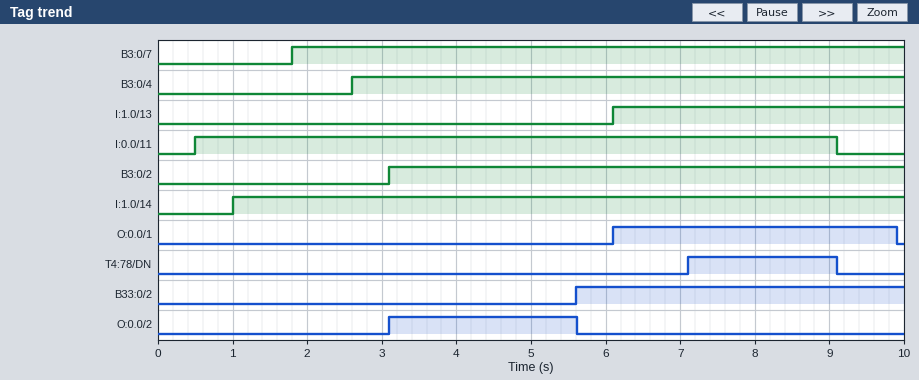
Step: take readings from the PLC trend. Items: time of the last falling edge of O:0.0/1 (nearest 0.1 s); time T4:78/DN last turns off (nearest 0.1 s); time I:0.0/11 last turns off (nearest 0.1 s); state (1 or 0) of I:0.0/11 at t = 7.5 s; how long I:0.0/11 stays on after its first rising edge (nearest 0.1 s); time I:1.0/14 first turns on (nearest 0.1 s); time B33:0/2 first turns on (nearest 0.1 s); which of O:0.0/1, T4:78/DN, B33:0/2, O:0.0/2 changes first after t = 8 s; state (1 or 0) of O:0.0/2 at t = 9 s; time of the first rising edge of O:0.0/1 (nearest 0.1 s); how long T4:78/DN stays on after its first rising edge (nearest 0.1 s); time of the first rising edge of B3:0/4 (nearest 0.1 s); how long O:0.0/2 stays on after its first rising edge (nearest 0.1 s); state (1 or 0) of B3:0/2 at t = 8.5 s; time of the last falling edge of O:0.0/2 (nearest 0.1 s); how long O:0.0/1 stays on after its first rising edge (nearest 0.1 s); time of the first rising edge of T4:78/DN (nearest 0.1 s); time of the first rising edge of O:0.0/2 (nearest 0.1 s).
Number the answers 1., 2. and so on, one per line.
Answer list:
1. 9.9 s
2. 9.1 s
3. 9.1 s
4. 1
5. 8.6 s
6. 1.0 s
7. 5.6 s
8. T4:78/DN
9. 0
10. 6.1 s
11. 2.0 s
12. 2.6 s
13. 2.5 s
14. 1
15. 5.6 s
16. 3.8 s
17. 7.1 s
18. 3.1 s
